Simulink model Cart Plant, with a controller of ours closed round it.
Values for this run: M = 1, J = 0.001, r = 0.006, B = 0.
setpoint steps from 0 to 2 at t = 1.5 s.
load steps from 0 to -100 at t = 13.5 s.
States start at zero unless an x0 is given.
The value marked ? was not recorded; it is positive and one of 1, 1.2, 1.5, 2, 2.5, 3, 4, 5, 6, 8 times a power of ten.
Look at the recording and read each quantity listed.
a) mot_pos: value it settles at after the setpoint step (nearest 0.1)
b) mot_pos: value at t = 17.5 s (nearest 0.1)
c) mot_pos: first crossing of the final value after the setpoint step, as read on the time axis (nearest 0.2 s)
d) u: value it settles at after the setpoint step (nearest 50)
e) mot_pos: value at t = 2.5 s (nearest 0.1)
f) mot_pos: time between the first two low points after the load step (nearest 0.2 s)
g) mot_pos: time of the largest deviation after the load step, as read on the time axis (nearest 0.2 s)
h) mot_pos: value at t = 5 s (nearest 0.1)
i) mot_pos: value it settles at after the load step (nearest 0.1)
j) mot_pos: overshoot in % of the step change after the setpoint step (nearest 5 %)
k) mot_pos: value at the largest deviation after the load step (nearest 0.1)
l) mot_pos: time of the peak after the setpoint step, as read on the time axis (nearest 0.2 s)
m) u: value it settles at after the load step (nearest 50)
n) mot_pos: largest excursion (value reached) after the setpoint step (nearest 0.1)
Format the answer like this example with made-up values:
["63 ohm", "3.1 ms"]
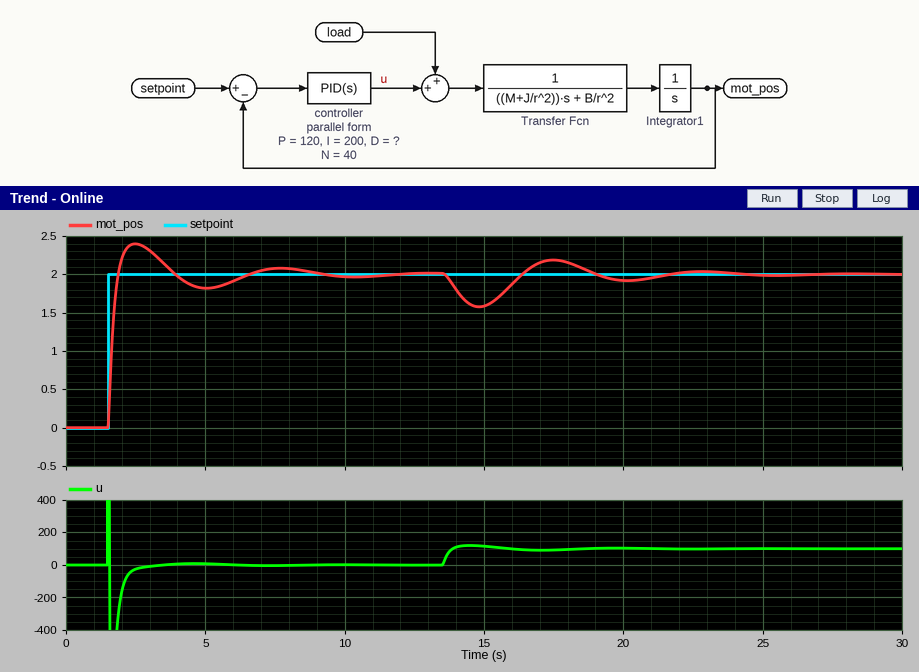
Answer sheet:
["2.0", "2.2", "1.8 s", "0", "2.4", "5.4 s", "14.8 s", "1.8", "2.0", "20 %", "1.6", "2.4 s", "100", "2.4"]
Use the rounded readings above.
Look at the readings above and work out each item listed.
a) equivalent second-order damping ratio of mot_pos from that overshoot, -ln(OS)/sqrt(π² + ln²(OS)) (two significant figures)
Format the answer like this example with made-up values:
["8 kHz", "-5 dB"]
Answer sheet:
["0.46"]
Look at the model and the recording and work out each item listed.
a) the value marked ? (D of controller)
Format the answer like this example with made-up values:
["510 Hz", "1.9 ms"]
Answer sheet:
["150"]
